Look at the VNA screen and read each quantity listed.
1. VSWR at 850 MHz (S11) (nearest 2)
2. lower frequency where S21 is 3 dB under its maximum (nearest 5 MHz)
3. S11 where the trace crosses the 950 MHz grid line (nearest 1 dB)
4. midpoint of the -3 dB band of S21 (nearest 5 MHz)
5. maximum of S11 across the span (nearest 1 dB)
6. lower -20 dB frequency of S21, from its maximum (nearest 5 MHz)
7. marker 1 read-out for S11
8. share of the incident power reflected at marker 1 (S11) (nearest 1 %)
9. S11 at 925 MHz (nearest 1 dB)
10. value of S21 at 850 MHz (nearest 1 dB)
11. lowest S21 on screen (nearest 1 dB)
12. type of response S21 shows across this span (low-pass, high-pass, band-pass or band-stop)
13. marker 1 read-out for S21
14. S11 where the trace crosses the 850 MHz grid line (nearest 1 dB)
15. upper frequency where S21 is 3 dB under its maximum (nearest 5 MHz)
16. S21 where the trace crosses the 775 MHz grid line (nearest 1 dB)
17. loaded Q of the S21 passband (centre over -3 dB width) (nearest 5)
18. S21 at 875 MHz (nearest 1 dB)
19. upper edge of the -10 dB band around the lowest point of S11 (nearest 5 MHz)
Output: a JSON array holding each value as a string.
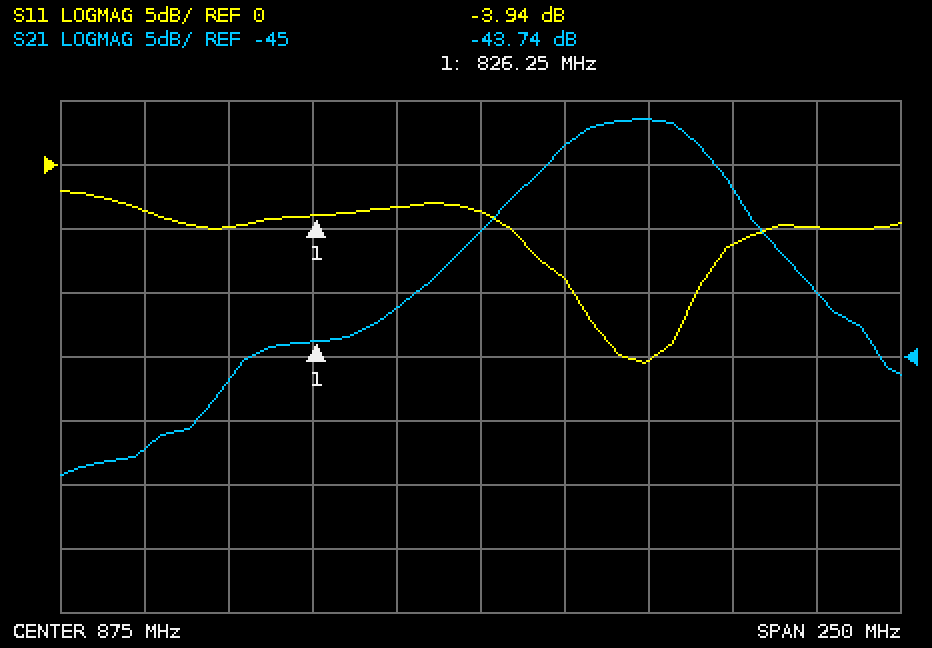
["6", "895 MHz", "-6 dB", "920 MHz", "-2 dB", "800 MHz", "-3.94 dB", "40 %", "-15 dB", "-41 dB", "-54 dB", "band-pass", "-43.74 dB", "-3 dB", "945 MHz", "-52 dB", "20", "-35 dB", "940 MHz"]
